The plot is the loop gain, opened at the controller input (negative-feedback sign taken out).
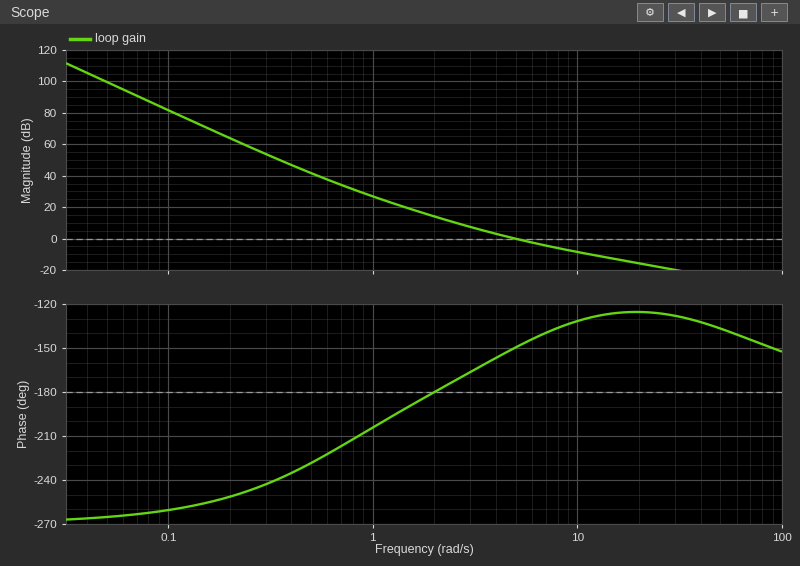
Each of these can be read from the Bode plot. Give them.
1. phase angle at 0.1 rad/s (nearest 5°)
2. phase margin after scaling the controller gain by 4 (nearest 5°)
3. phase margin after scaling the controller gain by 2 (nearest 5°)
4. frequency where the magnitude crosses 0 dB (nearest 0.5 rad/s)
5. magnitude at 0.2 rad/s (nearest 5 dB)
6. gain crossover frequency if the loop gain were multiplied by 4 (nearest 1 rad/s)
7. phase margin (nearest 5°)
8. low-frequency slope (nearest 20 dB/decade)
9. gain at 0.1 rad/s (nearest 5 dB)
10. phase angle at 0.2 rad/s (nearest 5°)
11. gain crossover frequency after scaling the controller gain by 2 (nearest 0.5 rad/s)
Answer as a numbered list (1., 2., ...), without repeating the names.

1. -260°
2. 55°
3. 45°
4. 5.0 rad/s
5. 65 dB
6. 14 rad/s
7. 30°
8. -60 dB/decade
9. 80 dB
10. -250°
11. 8.0 rad/s
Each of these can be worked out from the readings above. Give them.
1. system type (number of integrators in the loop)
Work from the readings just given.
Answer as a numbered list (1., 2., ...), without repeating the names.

1. 3
